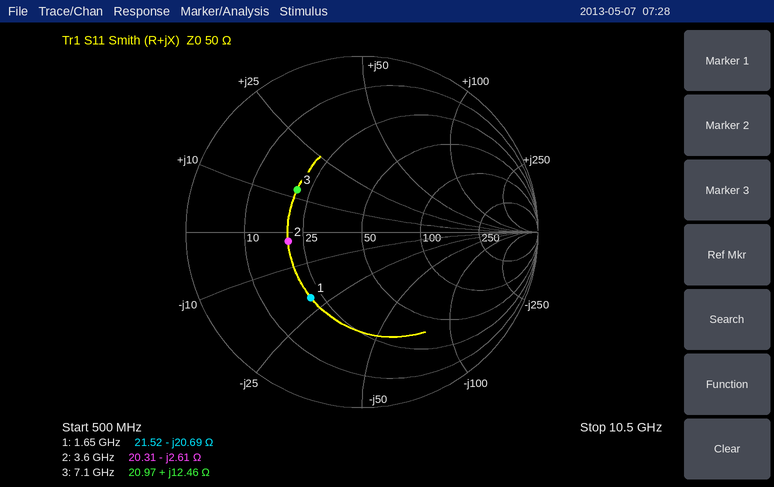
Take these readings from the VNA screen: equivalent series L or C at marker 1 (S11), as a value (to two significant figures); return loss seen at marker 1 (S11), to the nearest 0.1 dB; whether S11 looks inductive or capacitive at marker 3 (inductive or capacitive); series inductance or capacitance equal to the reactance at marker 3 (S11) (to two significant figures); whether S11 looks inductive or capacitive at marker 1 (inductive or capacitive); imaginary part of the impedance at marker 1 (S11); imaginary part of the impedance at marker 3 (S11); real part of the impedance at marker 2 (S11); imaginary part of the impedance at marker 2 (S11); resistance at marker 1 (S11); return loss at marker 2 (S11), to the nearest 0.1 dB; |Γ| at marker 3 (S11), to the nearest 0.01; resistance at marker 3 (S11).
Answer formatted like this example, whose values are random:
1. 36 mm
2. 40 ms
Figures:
1. 4.7 pF
2. 6.5 dB
3. inductive
4. 280 pH
5. capacitive
6. -20.69 Ω
7. +12.46 Ω
8. 20.31 Ω
9. -2.61 Ω
10. 21.52 Ω
11. 7.5 dB
12. 0.44
13. 20.97 Ω
